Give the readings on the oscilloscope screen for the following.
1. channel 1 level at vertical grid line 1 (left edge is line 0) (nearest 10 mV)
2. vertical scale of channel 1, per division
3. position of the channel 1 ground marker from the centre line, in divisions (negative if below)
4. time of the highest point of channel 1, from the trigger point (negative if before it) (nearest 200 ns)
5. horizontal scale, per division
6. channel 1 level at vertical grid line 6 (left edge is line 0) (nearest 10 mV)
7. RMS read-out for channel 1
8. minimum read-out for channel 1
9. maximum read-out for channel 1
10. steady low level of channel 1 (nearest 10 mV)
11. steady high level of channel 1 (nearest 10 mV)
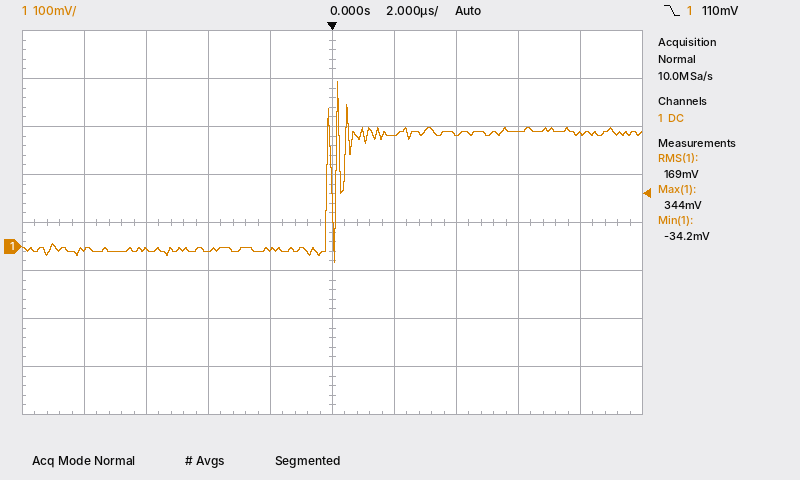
-10 mV
100 mV
-0.5 div
+200 ns
2 µs
230 mV
169 mV
-34.2 mV
344 mV
-10 mV
240 mV
